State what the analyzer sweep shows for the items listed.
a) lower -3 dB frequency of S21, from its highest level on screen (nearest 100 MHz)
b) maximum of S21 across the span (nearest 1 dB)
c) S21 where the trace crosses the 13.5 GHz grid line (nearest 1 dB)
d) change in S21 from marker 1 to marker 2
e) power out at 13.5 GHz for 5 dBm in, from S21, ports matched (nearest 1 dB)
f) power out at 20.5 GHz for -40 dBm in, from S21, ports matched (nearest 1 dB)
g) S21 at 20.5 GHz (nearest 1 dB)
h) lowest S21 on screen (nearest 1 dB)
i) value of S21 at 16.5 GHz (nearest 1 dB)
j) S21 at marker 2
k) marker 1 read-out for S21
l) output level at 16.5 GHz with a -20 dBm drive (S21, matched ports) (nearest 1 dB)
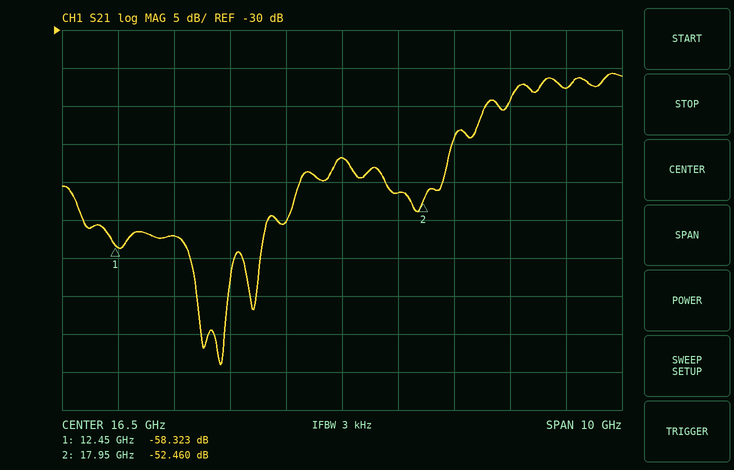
19.5 GHz
-36 dB
-57 dB
5.863 dB
-52 dBm
-78 dBm
-38 dB
-74 dB
-47 dB
-52.460 dB
-58.323 dB
-67 dBm
